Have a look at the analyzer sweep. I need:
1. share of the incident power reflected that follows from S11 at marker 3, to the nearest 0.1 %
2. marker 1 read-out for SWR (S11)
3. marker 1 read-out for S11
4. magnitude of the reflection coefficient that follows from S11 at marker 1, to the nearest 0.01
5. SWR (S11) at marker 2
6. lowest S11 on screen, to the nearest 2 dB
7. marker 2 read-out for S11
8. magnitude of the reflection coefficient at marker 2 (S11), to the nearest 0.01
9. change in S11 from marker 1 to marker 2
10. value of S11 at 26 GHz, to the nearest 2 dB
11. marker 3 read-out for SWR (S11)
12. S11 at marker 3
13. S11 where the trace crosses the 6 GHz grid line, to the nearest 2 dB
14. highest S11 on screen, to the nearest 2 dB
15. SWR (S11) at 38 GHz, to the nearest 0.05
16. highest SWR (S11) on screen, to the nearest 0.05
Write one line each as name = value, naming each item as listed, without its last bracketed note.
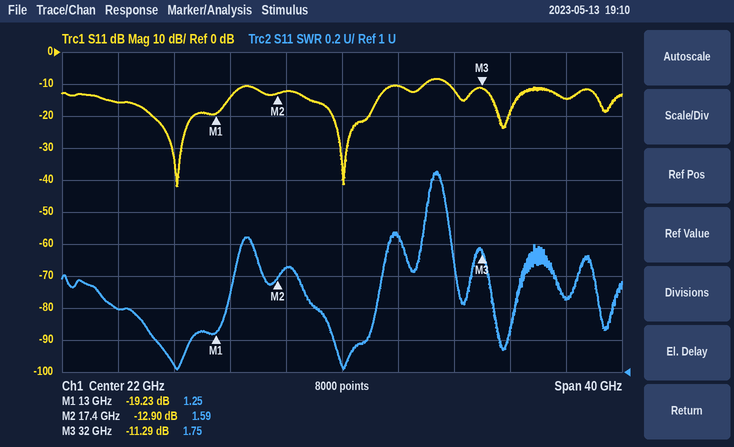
share of the incident power reflected that follows from S11 at marker 3, to the nearest 0.1 % = 7.4 %
marker 1 read-out for SWR = 1.25
marker 1 read-out for S11 = -19.23 dB
magnitude of the reflection coefficient that follows from S11 at marker 1, to the nearest 0.01 = 0.11
SWR (S11) at marker 2 = 1.59
lowest S11 on screen, to the nearest 2 dB = -42 dB
marker 2 read-out for S11 = -12.90 dB
magnitude of the reflection coefficient at marker 2 (S11), to the nearest 0.01 = 0.23
change in S11 from marker 1 to marker 2 = 6.33 dB
value of S11 at 26 GHz, to the nearest 2 dB = -10 dB
marker 3 read-out for SWR = 1.75
S11 at marker 3 = -11.29 dB
S11 where the trace crosses the 6 GHz grid line, to the nearest 2 dB = -16 dB
highest S11 on screen, to the nearest 2 dB = -8 dB
SWR (S11) at 38 GHz, to the nearest 0.05 = 1.45
highest SWR (S11) on screen, to the nearest 0.05 = 2.25
